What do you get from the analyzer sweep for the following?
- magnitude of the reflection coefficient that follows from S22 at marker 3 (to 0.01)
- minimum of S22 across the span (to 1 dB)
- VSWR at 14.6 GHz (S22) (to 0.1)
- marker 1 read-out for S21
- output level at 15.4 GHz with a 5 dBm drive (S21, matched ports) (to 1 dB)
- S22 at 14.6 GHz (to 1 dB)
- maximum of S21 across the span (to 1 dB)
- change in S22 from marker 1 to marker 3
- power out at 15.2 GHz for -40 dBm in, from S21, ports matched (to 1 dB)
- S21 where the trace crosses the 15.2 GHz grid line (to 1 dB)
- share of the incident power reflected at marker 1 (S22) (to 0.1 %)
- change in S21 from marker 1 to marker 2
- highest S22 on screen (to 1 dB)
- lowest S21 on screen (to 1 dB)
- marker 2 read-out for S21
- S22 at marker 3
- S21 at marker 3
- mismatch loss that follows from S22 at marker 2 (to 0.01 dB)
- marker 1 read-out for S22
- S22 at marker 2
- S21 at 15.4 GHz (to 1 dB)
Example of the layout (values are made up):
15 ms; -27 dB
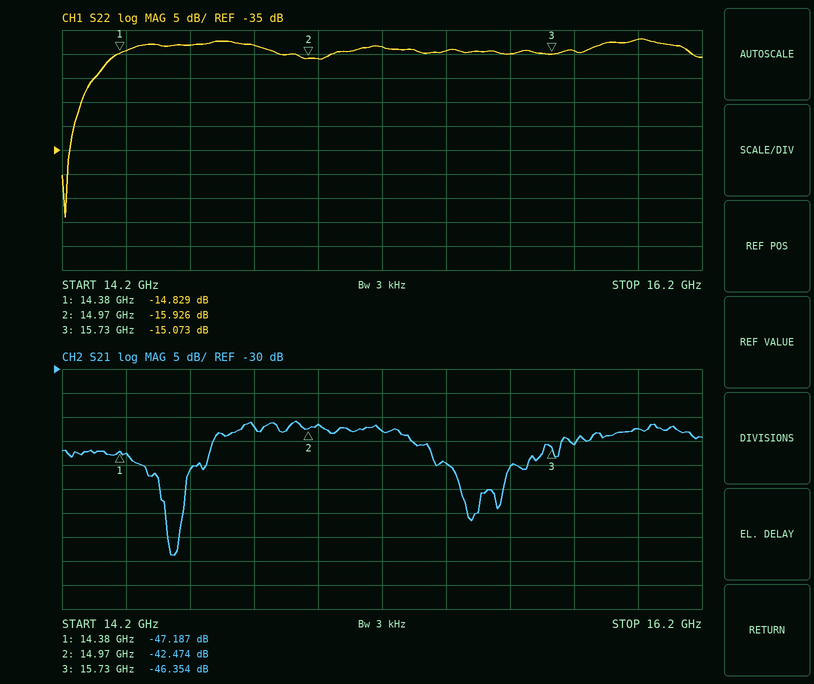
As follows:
0.18; -49 dB; 1.6; -47.187 dB; -45 dBm; -13 dB; -41 dB; -0.244 dB; -83 dBm; -43 dB; 3.3 %; 4.713 dB; -12 dB; -69 dB; -42.474 dB; -15.073 dB; -46.354 dB; 0.11 dB; -14.829 dB; -15.926 dB; -50 dB
